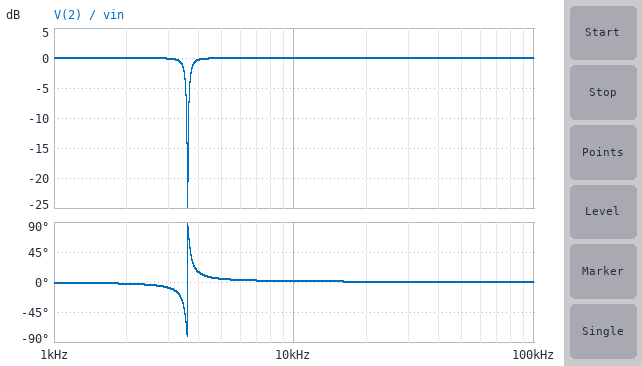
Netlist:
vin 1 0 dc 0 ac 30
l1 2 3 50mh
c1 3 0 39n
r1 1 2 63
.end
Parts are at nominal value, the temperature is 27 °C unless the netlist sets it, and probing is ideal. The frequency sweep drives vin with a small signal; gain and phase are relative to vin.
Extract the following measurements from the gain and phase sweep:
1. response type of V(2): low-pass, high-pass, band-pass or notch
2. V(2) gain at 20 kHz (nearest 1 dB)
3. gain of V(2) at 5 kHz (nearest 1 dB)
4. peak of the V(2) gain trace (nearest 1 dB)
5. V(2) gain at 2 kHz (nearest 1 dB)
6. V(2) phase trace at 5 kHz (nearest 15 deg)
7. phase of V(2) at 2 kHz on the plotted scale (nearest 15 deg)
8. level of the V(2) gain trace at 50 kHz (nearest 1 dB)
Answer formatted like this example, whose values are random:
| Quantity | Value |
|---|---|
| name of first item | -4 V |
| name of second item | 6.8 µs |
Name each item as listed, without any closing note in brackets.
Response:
| Quantity | Value |
|---|---|
| response type of V(2): low-pass, high-pass, band-pass or notch | notch |
| V(2) gain at 20 kHz | 0 dB |
| gain of V(2) at 5 kHz | 0 dB |
| peak of the V(2) gain trace | 0 dB |
| V(2) gain at 2 kHz | 0 dB |
| V(2) phase trace at 5 kHz | 0 deg |
| phase of V(2) at 2 kHz on the plotted scale | 0 deg |
| level of the V(2) gain trace at 50 kHz | 0 dB |
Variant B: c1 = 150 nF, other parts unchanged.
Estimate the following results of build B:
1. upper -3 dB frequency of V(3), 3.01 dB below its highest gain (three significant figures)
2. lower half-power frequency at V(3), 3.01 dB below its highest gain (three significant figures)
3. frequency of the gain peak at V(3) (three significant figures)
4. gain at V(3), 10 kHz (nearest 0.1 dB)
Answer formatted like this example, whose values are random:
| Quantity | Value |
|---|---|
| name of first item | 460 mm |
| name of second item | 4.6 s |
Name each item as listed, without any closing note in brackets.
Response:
| Quantity | Value |
|---|---|
| upper -3 dB frequency of V(3), 3.01 dB below its highest gain | 1.93 kHz |
| lower half-power frequency at V(3), 3.01 dB below its highest gain | 1.73 kHz |
| frequency of the gain peak at V(3) | 1.83 kHz |
| gain at V(3), 10 kHz | -29.1 dB |
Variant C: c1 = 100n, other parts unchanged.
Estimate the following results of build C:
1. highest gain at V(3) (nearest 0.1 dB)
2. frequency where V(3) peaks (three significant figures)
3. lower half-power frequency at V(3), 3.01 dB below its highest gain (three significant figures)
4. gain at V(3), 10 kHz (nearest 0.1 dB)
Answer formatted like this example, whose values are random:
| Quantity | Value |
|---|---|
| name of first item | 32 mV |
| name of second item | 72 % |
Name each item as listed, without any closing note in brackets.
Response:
| Quantity | Value |
|---|---|
| highest gain at V(3) | 21.0 dB |
| frequency where V(3) peaks | 2.25 kHz |
| lower half-power frequency at V(3), 3.01 dB below its highest gain | 2.14 kHz |
| gain at V(3), 10 kHz | -25.5 dB |
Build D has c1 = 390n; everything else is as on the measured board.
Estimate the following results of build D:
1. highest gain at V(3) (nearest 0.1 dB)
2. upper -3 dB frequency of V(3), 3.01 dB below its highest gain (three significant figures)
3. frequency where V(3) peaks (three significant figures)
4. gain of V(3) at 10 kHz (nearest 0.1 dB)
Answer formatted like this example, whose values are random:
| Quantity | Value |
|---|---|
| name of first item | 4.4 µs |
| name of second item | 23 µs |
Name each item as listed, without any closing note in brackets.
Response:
| Quantity | Value |
|---|---|
| highest gain at V(3) | 15.1 dB |
| upper -3 dB frequency of V(3), 3.01 dB below its highest gain | 1.23 kHz |
| frequency where V(3) peaks | 1.13 kHz |
| gain of V(3) at 10 kHz | -37.6 dB |
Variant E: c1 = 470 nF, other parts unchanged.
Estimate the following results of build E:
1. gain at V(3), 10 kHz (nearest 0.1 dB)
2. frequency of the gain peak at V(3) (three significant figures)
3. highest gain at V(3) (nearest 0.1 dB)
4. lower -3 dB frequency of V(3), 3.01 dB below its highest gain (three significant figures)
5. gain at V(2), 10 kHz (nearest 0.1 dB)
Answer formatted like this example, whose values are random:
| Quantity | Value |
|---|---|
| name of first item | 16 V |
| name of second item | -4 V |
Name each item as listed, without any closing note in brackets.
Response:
| Quantity | Value |
|---|---|
| gain at V(3), 10 kHz | -39.3 dB |
| frequency of the gain peak at V(3) | 1.03 kHz |
| highest gain at V(3) | 14.3 dB |
| lower -3 dB frequency of V(3), 3.01 dB below its highest gain | 922 Hz |
| gain at V(2), 10 kHz | 0 dB |
